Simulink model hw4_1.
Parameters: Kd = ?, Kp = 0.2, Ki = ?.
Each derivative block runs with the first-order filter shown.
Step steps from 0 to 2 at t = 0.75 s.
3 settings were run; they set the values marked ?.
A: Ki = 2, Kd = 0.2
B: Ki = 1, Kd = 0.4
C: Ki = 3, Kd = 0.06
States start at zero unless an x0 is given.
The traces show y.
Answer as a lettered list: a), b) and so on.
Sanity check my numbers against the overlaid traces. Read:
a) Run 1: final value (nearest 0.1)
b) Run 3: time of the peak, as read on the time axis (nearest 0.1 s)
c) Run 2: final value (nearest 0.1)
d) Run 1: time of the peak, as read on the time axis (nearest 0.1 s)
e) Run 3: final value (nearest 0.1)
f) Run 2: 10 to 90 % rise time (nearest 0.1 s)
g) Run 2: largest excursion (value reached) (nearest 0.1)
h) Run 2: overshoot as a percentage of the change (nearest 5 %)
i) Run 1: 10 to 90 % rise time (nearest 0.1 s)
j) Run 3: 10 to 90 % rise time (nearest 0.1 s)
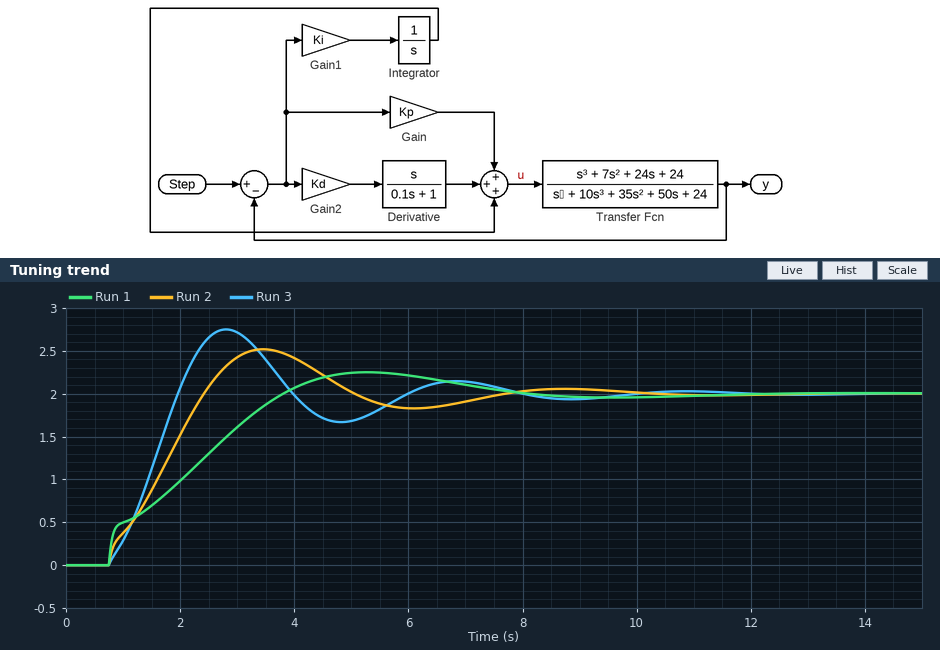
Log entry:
a) 2.0
b) 2.8 s
c) 2.0
d) 5.3 s
e) 2.0
f) 1.4 s
g) 2.5
h) 25 %
i) 2.6 s
j) 0.9 s
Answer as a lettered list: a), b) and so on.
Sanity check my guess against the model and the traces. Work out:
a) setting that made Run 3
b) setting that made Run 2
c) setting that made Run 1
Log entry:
a) C
b) A
c) B
